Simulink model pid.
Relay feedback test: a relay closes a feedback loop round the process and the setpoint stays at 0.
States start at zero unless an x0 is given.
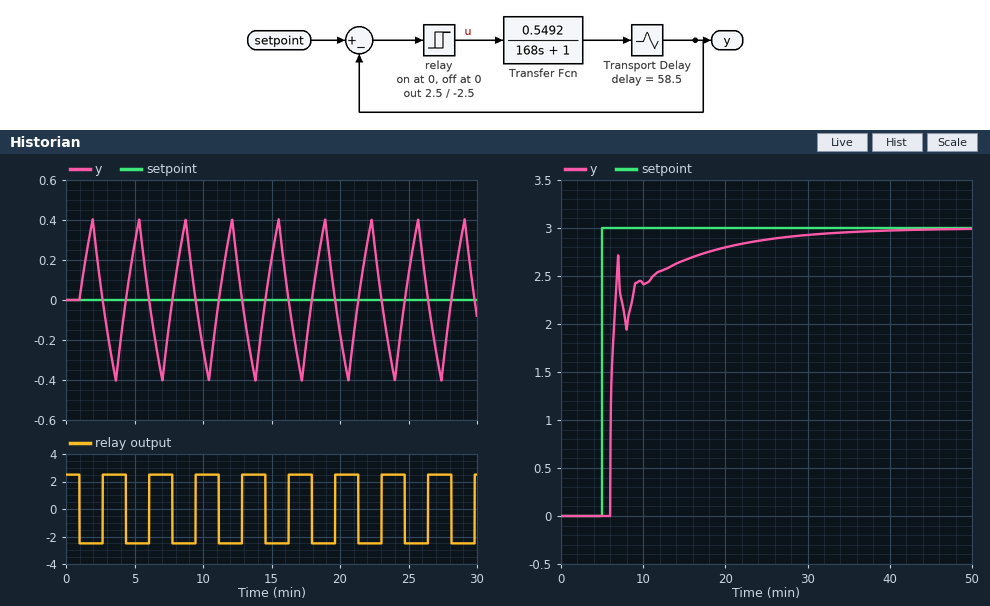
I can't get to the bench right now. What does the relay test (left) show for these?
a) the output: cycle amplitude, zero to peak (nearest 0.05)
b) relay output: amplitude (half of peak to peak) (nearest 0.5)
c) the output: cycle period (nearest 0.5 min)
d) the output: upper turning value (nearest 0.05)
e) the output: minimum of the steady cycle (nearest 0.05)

0.40
2.5
3.5 min
0.40
-0.40
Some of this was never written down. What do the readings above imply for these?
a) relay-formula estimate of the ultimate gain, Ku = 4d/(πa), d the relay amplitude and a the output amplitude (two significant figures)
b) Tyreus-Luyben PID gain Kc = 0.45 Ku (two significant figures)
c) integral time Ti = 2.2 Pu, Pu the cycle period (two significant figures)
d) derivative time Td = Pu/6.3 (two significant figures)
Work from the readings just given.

8.0
3.6
7.7 min
0.56 min
